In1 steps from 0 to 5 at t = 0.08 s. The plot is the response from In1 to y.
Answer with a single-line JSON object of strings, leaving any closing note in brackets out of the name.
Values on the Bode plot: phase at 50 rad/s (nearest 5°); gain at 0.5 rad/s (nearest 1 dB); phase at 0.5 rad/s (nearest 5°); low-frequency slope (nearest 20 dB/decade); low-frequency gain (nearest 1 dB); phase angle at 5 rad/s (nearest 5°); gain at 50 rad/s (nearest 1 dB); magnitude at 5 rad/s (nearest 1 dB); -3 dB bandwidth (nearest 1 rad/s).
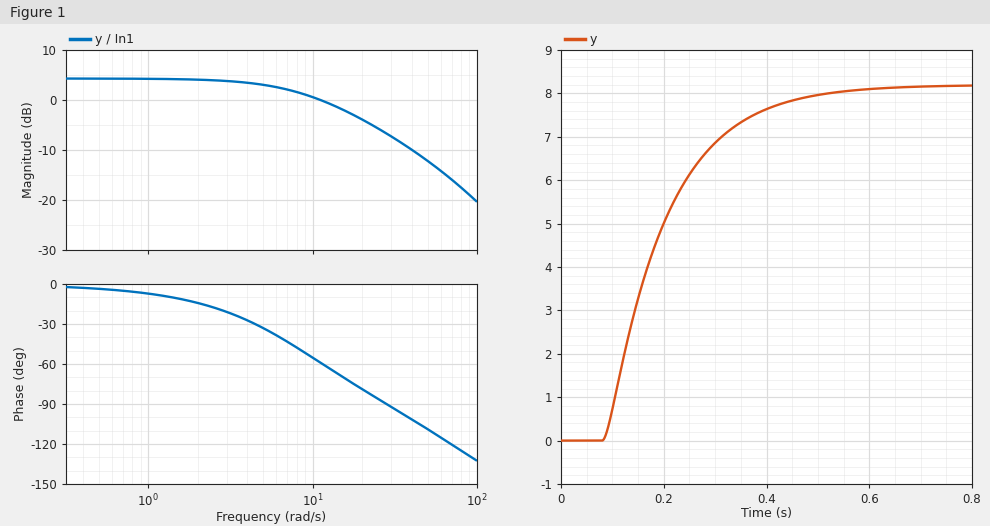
{"phase at 50 rad/s": "-110°", "gain at 0.5 rad/s": "4 dB", "phase at 0.5 rad/s": "-5°", "low-frequency slope": "0 dB/decade", "low-frequency gain": "4 dB", "phase angle at 5 rad/s": "-35°", "gain at 50 rad/s": "-12 dB", "magnitude at 5 rad/s": "3 dB", "-3 dB bandwidth": "9 rad/s"}
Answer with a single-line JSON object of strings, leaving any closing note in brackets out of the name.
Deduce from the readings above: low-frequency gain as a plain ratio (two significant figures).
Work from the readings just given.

{"low-frequency gain as a plain ratio": "1.6"}
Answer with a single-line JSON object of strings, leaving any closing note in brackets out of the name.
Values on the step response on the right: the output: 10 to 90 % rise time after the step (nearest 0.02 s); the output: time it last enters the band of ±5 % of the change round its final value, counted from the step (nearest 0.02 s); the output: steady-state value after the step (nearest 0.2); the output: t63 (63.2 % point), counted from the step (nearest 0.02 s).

{"the output: 10 to 90 % rise time after the step": "0.26 s", "the output: time it last enters the band of ±5 % of the change round its final value, counted from the step": "0.36 s", "the output: steady-state value after the step": "8.2", "the output: t63 (63.2 % point), counted from the step": "0.12 s"}
